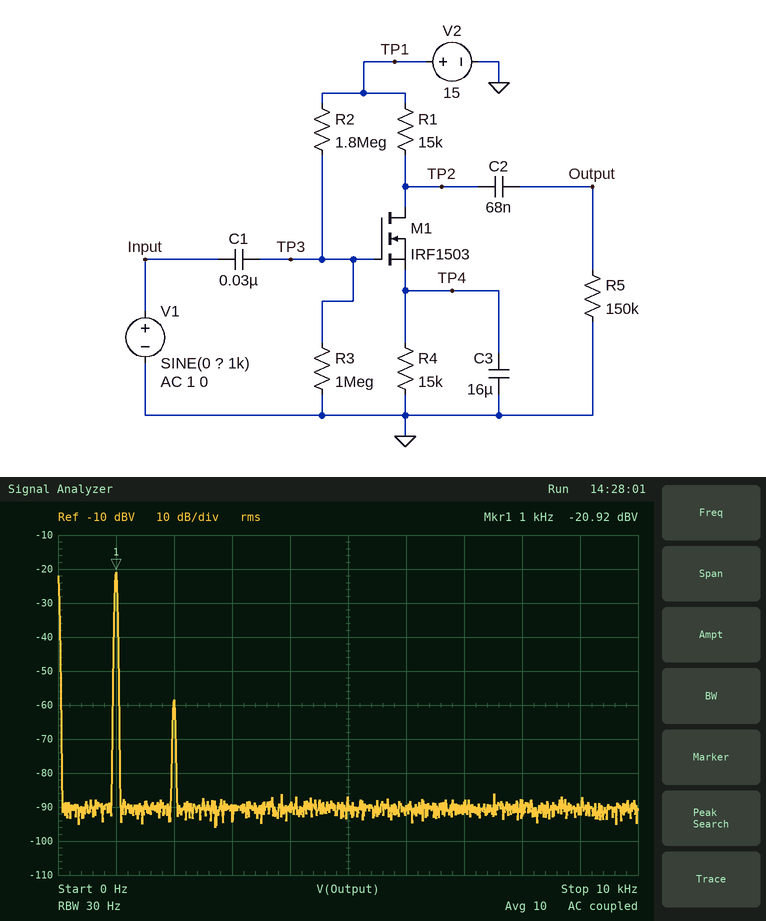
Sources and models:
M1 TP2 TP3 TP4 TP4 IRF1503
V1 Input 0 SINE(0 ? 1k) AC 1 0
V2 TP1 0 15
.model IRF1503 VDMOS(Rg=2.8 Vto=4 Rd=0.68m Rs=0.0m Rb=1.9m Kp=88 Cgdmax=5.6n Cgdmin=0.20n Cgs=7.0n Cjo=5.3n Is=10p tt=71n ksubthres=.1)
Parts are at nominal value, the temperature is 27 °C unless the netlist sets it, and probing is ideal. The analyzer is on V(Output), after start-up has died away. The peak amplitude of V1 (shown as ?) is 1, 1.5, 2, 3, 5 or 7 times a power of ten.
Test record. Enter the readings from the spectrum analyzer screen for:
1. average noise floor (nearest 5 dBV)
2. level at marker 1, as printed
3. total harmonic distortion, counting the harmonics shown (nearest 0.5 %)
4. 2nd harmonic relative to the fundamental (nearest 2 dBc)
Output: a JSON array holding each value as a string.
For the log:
["-90 dBV", "-20.92 dBV", "1.5 %", "-38 dBc"]
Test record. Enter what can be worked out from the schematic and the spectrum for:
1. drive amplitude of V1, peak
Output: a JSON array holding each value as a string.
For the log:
["7 mV"]
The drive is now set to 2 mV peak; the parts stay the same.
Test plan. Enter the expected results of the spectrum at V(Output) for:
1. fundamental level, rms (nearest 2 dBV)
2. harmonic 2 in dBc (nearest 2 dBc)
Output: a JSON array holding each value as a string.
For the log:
["-32 dBV", "-48 dBc"]
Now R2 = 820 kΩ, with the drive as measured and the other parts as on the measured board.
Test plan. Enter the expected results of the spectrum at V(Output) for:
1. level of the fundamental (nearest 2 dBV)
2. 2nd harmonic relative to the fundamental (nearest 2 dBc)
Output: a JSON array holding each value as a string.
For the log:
["-20 dBV", "-44 dBc"]
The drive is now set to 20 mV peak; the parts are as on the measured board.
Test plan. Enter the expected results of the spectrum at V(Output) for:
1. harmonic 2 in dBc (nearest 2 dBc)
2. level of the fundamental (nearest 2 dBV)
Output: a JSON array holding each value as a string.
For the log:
["-28 dBc", "-12 dBV"]
